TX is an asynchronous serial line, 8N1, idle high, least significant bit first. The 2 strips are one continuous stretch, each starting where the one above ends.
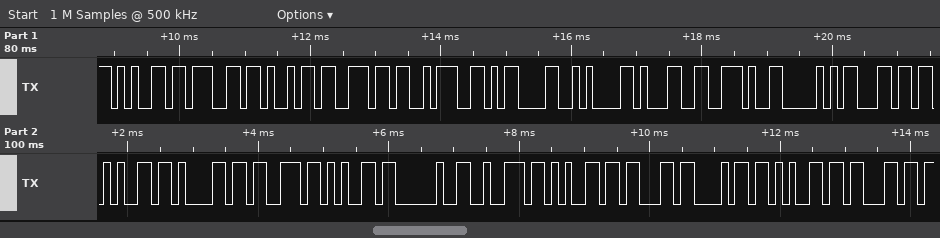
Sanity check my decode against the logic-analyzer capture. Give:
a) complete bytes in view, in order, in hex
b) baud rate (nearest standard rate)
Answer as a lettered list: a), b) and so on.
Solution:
a) 65 67 69 6E 3A 0D 0A 31 2E 50 6C 65 61 73 65 20 72 65 63 68 65 63
b) 9600 baud
